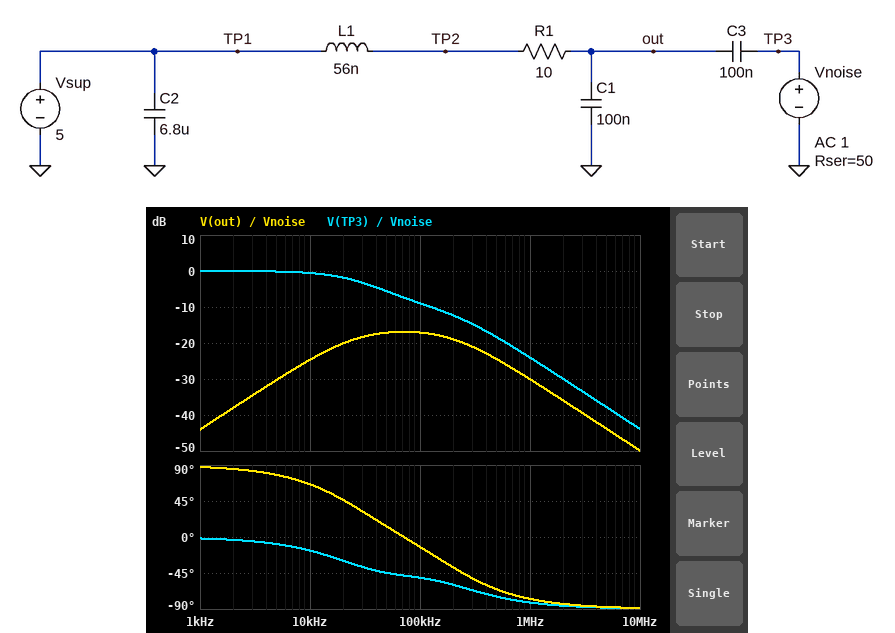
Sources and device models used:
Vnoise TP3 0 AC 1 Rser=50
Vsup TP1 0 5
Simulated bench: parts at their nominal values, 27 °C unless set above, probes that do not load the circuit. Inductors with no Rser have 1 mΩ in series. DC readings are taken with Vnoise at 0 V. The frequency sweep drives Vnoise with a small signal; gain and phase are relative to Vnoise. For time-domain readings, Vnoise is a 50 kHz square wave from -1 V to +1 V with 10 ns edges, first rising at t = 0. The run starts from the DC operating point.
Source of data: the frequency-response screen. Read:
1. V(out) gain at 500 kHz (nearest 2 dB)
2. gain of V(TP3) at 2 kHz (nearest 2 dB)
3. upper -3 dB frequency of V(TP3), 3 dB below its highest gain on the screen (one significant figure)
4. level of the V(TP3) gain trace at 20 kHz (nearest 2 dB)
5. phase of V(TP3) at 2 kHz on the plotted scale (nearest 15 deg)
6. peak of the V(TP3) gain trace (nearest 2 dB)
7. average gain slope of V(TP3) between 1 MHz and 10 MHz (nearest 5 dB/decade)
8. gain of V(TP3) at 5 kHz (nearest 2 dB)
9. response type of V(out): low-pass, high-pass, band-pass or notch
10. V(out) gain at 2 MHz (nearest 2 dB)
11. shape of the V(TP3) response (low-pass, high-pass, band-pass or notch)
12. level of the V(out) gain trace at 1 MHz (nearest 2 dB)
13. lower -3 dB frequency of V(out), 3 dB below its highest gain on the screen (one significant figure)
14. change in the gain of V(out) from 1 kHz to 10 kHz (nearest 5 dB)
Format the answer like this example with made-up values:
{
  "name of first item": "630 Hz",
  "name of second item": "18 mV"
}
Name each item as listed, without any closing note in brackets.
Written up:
{
  "V(out) gain at 500 kHz": "-24 dB",
  "gain of V(TP3) at 2 kHz": "0 dB",
  "upper -3 dB frequency of V(TP3), 3 dB below its highest gain on the screen": "30 kHz",
  "level of the V(TP3) gain trace at 20 kHz": "-2 dB",
  "phase of V(TP3) at 2 kHz on the plotted scale": "0 deg",
  "peak of the V(TP3) gain trace": "0 dB",
  "average gain slope of V(TP3) between 1 MHz and 10 MHz": "-20 dB/decade",
  "gain of V(TP3) at 5 kHz": "0 dB",
  "response type of V(out): low-pass, high-pass, band-pass or notch": "band-pass",
  "V(out) gain at 2 MHz": "-36 dB",
  "shape of the V(TP3) response": "low-pass",
  "level of the V(out) gain trace at 1 MHz": "-30 dB",
  "lower -3 dB frequency of V(out), 3 dB below its highest gain on the screen": "20 kHz",
  "change in the gain of V(out) from 1 kHz to 10 kHz": "20 dB"
}
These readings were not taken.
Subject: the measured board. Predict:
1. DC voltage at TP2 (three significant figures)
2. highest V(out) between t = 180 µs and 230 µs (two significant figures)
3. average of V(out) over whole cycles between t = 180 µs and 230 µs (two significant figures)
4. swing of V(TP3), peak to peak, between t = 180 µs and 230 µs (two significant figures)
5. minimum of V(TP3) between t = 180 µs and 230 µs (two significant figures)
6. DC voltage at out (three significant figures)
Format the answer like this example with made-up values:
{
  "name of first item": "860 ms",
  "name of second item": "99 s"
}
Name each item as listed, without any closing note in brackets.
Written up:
{
  "DC voltage at TP2": "5.00 V",
  "highest V(out) between t = 180 µs and 230 µs": "5.2 V",
  "average of V(out) over whole cycles between t = 180 µs and 230 µs": "5.0 V",
  "swing of V(TP3), peak to peak, between t = 180 µs and 230 µs": "1.5 V",
  "minimum of V(TP3) between t = 180 µs and 230 µs": "-740 mV",
  "DC voltage at out": "5.00 V"
}
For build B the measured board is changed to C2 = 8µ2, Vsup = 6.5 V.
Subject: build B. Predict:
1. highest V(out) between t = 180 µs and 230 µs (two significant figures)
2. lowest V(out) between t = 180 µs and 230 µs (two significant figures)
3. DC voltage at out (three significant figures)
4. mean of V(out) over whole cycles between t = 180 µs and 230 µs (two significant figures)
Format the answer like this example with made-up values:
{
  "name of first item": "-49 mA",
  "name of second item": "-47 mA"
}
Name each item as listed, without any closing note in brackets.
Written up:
{
  "highest V(out) between t = 180 µs and 230 µs": "6.7 V",
  "lowest V(out) between t = 180 µs and 230 µs": "6.3 V",
  "DC voltage at out": "6.50 V",
  "mean of V(out) over whole cycles between t = 180 µs and 230 µs": "6.5 V"
}
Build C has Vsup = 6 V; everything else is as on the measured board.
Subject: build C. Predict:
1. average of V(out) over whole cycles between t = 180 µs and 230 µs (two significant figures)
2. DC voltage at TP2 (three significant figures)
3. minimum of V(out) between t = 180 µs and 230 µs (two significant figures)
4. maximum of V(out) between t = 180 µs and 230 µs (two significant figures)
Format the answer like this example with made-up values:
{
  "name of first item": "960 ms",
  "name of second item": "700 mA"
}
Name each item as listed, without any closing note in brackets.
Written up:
{
  "average of V(out) over whole cycles between t = 180 µs and 230 µs": "6.0 V",
  "DC voltage at TP2": "6.00 V",
  "minimum of V(out) between t = 180 µs and 230 µs": "5.8 V",
  "maximum of V(out) between t = 180 µs and 230 µs": "6.2 V"
}
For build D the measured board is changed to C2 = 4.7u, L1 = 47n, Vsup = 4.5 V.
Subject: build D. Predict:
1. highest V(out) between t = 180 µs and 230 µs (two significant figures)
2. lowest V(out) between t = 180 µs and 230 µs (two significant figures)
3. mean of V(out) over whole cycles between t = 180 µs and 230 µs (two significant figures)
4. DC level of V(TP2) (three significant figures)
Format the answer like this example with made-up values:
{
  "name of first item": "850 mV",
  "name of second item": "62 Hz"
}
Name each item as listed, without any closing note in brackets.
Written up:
{
  "highest V(out) between t = 180 µs and 230 µs": "4.7 V",
  "lowest V(out) between t = 180 µs and 230 µs": "4.3 V",
  "mean of V(out) over whole cycles between t = 180 µs and 230 µs": "4.5 V",
  "DC level of V(TP2)": "4.50 V"
}
